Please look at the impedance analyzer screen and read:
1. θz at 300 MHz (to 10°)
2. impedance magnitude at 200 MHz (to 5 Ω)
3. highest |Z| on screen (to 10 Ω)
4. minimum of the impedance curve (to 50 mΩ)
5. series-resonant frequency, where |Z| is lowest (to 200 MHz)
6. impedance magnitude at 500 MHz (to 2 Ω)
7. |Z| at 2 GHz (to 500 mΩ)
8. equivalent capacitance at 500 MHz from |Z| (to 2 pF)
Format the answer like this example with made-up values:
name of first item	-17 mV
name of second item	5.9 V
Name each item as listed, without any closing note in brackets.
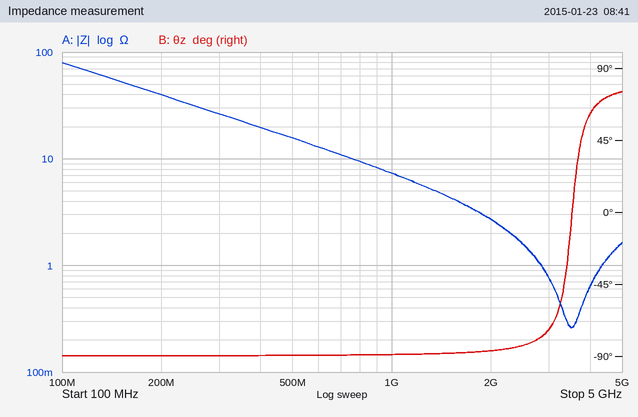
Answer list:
θz at 300 MHz	-90°
impedance magnitude at 200 MHz	40 Ω
highest |Z| on screen	80 Ω
minimum of the impedance curve	250 mΩ
series-resonant frequency, where |Z| is lowest	3.6 GHz
impedance magnitude at 500 MHz	16 Ω
|Z| at 2 GHz	2.5 Ω
equivalent capacitance at 500 MHz from |Z|	20 pF
